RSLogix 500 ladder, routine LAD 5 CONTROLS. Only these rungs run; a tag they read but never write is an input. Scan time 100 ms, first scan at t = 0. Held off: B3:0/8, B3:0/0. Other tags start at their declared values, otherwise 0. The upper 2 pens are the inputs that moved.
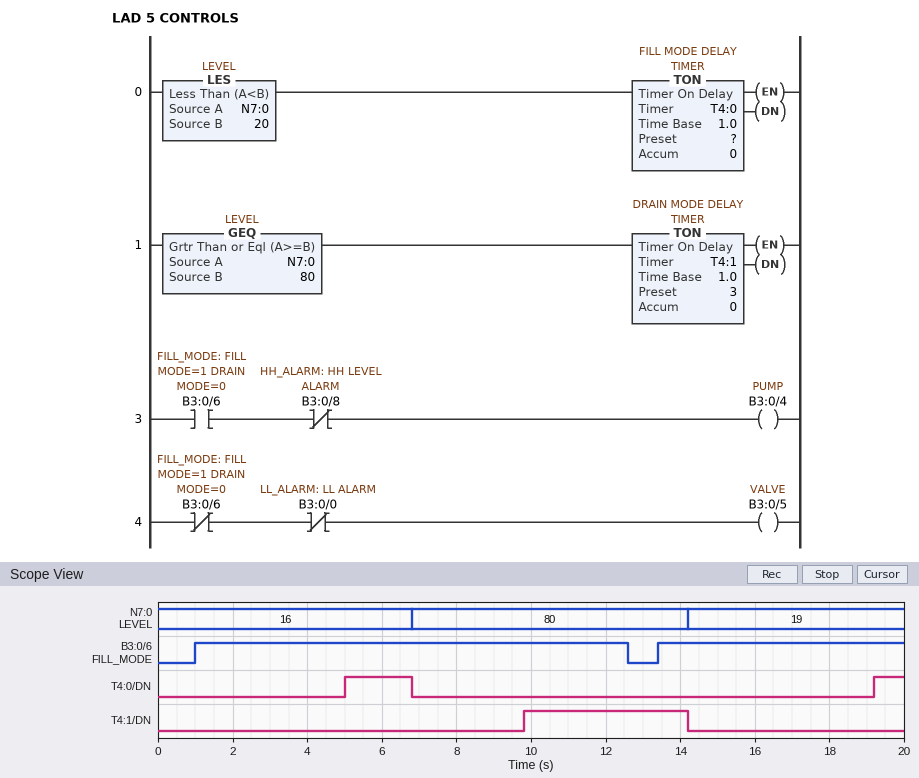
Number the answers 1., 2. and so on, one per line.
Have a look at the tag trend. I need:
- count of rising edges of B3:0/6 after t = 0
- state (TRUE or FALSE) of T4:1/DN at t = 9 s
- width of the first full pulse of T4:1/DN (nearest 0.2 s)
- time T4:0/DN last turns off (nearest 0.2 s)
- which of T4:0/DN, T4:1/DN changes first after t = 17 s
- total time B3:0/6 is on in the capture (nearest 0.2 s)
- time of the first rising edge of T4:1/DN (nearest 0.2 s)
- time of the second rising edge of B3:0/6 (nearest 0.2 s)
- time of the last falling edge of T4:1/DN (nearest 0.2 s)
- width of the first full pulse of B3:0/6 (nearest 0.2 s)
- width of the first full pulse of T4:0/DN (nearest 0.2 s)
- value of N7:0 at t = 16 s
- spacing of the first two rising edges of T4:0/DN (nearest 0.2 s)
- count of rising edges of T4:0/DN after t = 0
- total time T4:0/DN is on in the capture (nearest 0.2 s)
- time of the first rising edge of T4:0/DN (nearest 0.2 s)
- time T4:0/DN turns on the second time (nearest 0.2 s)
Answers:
1. 2
2. FALSE
3. 4.4 s
4. 6.8 s
5. T4:0/DN
6. 18.2 s
7. 9.8 s
8. 13.4 s
9. 14.2 s
10. 11.6 s
11. 1.8 s
12. 19
13. 14.2 s
14. 2
15. 2.6 s
16. 5.0 s
17. 19.2 s
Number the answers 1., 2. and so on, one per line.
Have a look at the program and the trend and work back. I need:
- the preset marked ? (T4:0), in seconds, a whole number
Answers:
1. 5 s
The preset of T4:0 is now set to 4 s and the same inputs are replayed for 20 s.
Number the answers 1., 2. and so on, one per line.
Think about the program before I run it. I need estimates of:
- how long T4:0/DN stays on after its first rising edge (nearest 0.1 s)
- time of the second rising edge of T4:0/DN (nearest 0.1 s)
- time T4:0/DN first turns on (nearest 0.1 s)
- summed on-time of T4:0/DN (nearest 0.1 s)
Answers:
1. 2.8 s
2. 18.2 s
3. 4.0 s
4. 4.6 s
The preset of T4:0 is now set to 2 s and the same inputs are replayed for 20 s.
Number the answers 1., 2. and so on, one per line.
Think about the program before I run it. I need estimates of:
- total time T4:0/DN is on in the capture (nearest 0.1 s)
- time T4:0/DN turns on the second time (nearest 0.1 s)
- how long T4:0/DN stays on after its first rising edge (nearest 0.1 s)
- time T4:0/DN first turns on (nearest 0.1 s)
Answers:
1. 8.6 s
2. 16.2 s
3. 4.8 s
4. 2.0 s
